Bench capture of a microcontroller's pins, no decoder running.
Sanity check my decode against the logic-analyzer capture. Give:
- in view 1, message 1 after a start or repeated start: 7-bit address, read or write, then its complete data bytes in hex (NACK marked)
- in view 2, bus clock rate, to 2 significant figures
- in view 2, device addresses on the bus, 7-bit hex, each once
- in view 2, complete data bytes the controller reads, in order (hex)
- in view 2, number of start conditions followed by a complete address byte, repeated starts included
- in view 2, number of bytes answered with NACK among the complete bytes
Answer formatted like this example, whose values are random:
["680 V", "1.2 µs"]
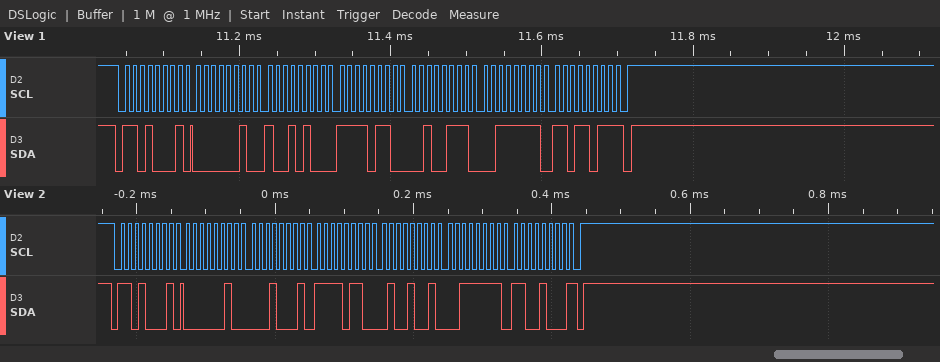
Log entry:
["0x68 read: 02 94 F6 27 3F DB NACK", "100 kHz", "0x68", "02 11 F6 49 3F C8", "1", "1"]
